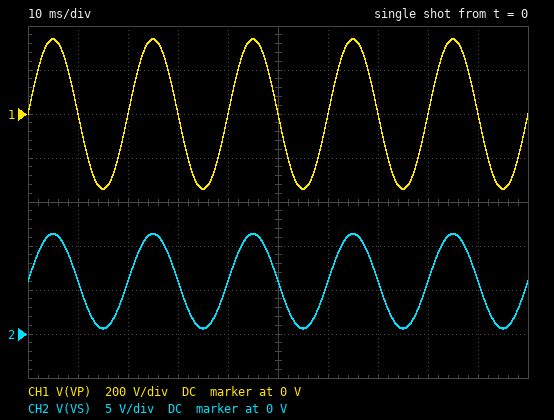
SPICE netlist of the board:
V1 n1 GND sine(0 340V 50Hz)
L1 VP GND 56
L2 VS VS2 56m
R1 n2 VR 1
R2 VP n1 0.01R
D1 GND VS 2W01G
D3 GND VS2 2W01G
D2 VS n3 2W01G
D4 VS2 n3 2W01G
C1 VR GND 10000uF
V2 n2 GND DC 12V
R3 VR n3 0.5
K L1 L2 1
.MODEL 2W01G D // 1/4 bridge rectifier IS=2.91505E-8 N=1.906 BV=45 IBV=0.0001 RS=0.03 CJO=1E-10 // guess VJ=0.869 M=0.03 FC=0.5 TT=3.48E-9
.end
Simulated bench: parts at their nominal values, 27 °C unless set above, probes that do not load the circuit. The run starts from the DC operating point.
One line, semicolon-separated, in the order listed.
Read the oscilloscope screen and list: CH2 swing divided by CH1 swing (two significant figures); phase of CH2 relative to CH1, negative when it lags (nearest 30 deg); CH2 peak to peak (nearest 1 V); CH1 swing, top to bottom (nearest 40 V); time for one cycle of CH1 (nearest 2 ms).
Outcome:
0.016; 0 deg; 11 V; 680 V; 20 ms
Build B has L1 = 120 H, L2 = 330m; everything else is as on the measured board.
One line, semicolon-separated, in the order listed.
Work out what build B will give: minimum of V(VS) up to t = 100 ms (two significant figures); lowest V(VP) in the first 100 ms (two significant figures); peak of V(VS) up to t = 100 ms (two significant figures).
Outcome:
-880 mV; -340 V; 17 V
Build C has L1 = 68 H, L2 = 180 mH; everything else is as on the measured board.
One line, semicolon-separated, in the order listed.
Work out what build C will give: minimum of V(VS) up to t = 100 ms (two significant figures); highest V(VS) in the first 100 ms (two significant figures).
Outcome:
-880 mV; 17 V
